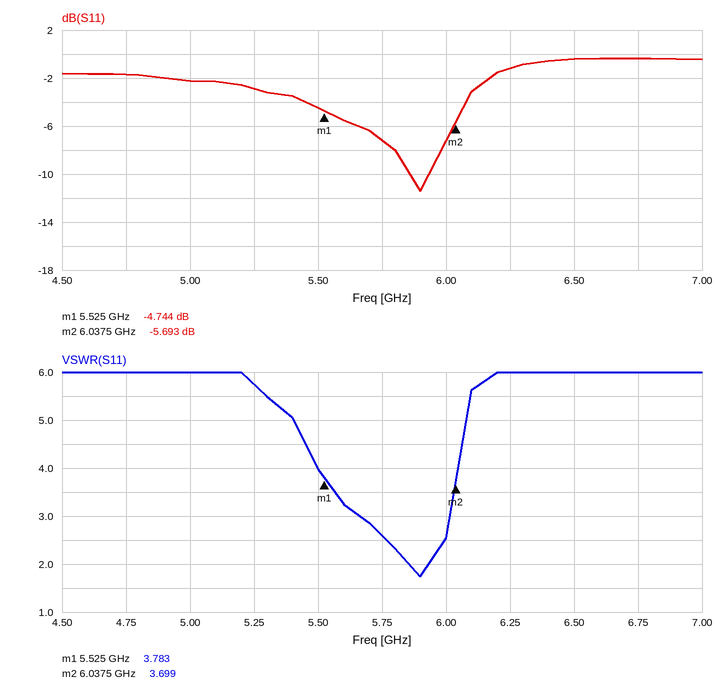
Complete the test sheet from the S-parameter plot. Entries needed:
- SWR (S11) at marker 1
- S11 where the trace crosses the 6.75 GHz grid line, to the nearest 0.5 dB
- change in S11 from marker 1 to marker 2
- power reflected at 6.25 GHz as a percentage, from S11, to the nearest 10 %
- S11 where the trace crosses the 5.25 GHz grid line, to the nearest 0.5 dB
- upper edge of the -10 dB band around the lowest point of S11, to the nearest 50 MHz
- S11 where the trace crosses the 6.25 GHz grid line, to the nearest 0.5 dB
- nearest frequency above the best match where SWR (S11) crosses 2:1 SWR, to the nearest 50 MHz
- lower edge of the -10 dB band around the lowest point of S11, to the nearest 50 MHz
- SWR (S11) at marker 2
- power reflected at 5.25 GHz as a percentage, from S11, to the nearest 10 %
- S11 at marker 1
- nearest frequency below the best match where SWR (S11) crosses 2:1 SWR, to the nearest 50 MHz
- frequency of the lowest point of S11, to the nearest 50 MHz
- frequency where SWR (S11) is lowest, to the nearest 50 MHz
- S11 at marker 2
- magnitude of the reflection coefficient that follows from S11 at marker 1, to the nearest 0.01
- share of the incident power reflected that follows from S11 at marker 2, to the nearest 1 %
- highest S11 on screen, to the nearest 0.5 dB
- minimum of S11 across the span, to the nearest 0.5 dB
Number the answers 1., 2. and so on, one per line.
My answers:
1. 3.783
2. -0.5 dB
3. -0.949 dB
4. 80 %
5. -3.0 dB
6. 5.95 GHz
7. -1.0 dB
8. 5.95 GHz
9. 5.85 GHz
10. 3.699
11. 50 %
12. -4.744 dB
13. 5.85 GHz
14. 5.90 GHz
15. 5.90 GHz
16. -5.693 dB
17. 0.58
18. 27 %
19. -0.5 dB
20. -11.5 dB
